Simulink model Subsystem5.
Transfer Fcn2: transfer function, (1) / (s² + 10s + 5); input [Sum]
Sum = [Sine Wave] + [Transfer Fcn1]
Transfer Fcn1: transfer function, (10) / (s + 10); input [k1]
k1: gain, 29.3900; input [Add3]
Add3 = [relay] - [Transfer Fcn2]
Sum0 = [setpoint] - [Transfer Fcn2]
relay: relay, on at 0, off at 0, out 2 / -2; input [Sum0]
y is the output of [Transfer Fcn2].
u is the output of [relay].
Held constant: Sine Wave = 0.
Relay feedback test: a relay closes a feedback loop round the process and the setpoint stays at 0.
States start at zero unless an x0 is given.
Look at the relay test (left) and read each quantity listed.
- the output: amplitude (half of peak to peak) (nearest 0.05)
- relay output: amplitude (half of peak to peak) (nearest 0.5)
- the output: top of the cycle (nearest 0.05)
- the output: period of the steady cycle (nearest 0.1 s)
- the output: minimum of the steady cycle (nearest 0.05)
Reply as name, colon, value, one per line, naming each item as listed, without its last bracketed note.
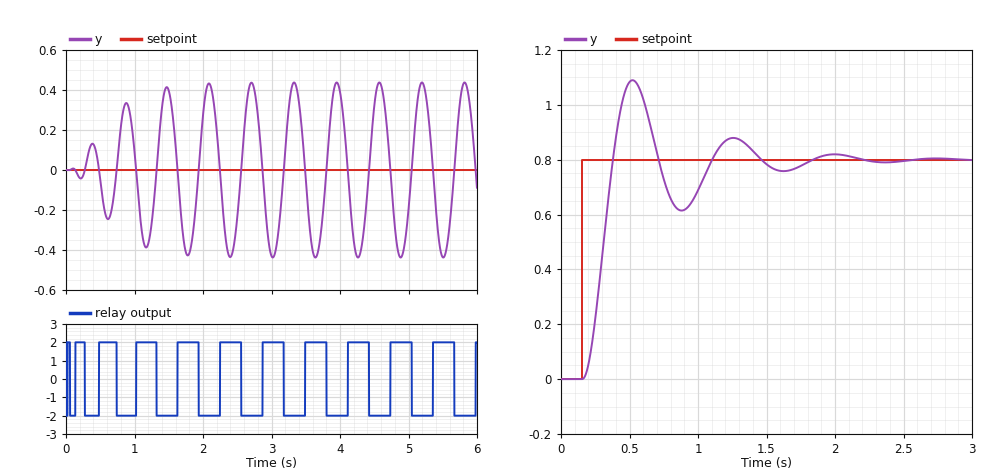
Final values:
the output: amplitude (half of peak to peak): 0.45
relay output: amplitude (half of peak to peak): 2.0
the output: top of the cycle: 0.45
the output: period of the steady cycle: 0.6 s
the output: minimum of the steady cycle: -0.45
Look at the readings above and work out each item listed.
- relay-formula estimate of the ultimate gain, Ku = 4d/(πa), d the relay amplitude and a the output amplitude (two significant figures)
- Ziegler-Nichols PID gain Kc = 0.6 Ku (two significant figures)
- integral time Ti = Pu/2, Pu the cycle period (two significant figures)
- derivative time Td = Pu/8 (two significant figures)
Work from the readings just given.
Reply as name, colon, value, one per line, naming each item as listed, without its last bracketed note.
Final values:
relay-formula estimate of the ultimate gain, Ku = 4d/(πa), d the relay amplitude and a the output amplitude: 5.7
Ziegler-Nichols PID gain Kc = 0.6 Ku: 3.4
integral time Ti = Pu/2, Pu the cycle period: 0.30 s
derivative time Td = Pu/8: 0.075 s
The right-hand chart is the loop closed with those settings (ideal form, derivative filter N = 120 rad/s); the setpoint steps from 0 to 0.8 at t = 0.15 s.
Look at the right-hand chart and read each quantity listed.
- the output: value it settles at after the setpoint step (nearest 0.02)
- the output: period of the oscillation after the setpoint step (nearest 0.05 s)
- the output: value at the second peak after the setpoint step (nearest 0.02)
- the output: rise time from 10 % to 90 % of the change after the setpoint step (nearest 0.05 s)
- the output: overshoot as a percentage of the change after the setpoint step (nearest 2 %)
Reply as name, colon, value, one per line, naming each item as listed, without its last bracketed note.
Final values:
the output: value it settles at after the setpoint step: 0.80
the output: period of the oscillation after the setpoint step: 0.75 s
the output: value at the second peak after the setpoint step: 0.88
the output: rise time from 10 % to 90 % of the change after the setpoint step: 0.15 s
the output: overshoot as a percentage of the change after the setpoint step: 36 %
